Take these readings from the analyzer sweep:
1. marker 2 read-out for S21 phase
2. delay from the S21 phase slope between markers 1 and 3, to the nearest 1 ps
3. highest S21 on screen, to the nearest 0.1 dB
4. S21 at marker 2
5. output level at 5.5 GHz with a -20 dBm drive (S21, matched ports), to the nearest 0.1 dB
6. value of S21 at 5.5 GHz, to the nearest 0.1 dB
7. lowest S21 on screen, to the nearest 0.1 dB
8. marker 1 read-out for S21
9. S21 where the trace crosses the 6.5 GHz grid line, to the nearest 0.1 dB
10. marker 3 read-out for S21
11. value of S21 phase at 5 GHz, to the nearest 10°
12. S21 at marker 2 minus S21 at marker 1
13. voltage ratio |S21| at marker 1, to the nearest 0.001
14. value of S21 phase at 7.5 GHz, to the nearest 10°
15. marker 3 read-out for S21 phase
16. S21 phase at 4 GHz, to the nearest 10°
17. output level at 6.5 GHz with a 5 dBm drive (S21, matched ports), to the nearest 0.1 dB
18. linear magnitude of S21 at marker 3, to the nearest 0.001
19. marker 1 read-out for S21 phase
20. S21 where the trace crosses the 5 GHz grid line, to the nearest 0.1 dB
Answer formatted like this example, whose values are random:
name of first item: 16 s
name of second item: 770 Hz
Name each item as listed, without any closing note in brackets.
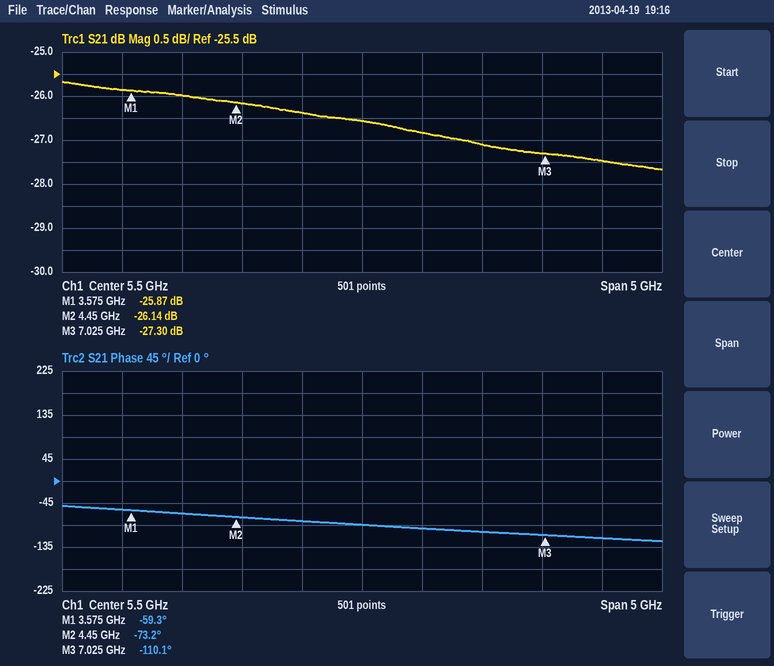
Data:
marker 2 read-out for S21 phase: -73.2°
delay from the S21 phase slope between markers 1 and 3, to the nearest 1 ps: 41 ps
highest S21 on screen, to the nearest 0.1 dB: -25.7 dB
S21 at marker 2: -26.14 dB
output level at 5.5 GHz with a -20 dBm drive (S21, matched ports), to the nearest 0.1 dB: -46.6 dBm
value of S21 at 5.5 GHz, to the nearest 0.1 dB: -26.6 dB
lowest S21 on screen, to the nearest 0.1 dB: -27.7 dB
marker 1 read-out for S21: -25.87 dB
S21 where the trace crosses the 6.5 GHz grid line, to the nearest 0.1 dB: -27.1 dB
marker 3 read-out for S21: -27.30 dB
value of S21 phase at 5 GHz, to the nearest 10°: -80°
S21 at marker 2 minus S21 at marker 1: -0.27 dB
voltage ratio |S21| at marker 1, to the nearest 0.001: 0.051
value of S21 phase at 7.5 GHz, to the nearest 10°: -120°
marker 3 read-out for S21 phase: -110.1°
S21 phase at 4 GHz, to the nearest 10°: -70°
output level at 6.5 GHz with a 5 dBm drive (S21, matched ports), to the nearest 0.1 dB: -22.1 dBm
linear magnitude of S21 at marker 3, to the nearest 0.001: 0.043
marker 1 read-out for S21 phase: -59.3°
S21 where the trace crosses the 5 GHz grid line, to the nearest 0.1 dB: -26.4 dB
